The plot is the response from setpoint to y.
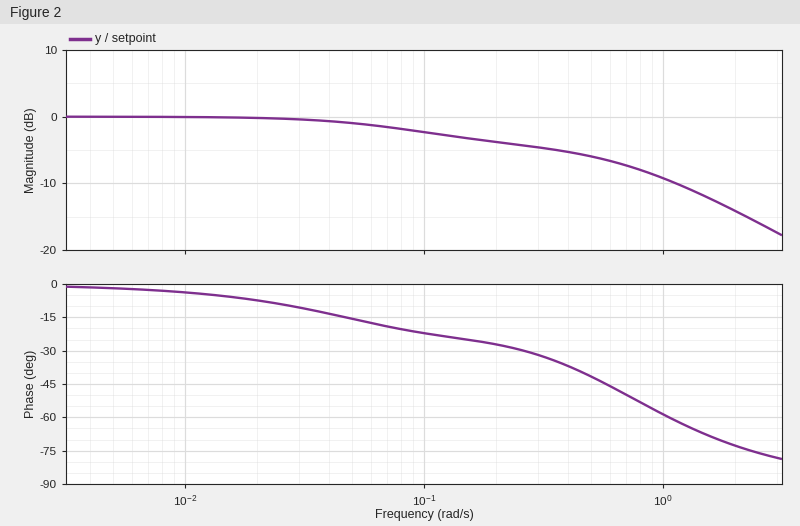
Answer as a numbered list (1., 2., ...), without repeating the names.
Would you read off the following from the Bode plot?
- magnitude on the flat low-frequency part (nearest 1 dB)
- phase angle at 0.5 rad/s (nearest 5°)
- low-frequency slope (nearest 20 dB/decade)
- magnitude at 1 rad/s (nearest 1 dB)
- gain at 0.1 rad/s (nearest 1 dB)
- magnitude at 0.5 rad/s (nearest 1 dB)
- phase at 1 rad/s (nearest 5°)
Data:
1. 0 dB
2. -40°
3. 0 dB/decade
4. -9 dB
5. -2 dB
6. -6 dB
7. -60°
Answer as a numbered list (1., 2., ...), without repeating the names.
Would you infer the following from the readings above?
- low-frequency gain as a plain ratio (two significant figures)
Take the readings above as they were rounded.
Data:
1. 1.0
